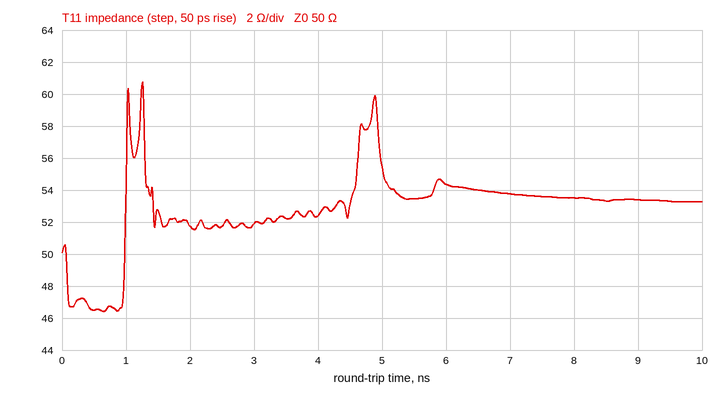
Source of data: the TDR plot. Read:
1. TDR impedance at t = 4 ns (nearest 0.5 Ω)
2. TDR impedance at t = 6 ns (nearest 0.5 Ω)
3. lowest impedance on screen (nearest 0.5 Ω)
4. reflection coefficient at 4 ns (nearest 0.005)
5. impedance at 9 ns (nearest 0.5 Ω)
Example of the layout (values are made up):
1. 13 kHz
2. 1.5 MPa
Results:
1. 52.5 Ω
2. 54.5 Ω
3. 46.5 Ω
4. +0.025
5. 53.5 Ω
